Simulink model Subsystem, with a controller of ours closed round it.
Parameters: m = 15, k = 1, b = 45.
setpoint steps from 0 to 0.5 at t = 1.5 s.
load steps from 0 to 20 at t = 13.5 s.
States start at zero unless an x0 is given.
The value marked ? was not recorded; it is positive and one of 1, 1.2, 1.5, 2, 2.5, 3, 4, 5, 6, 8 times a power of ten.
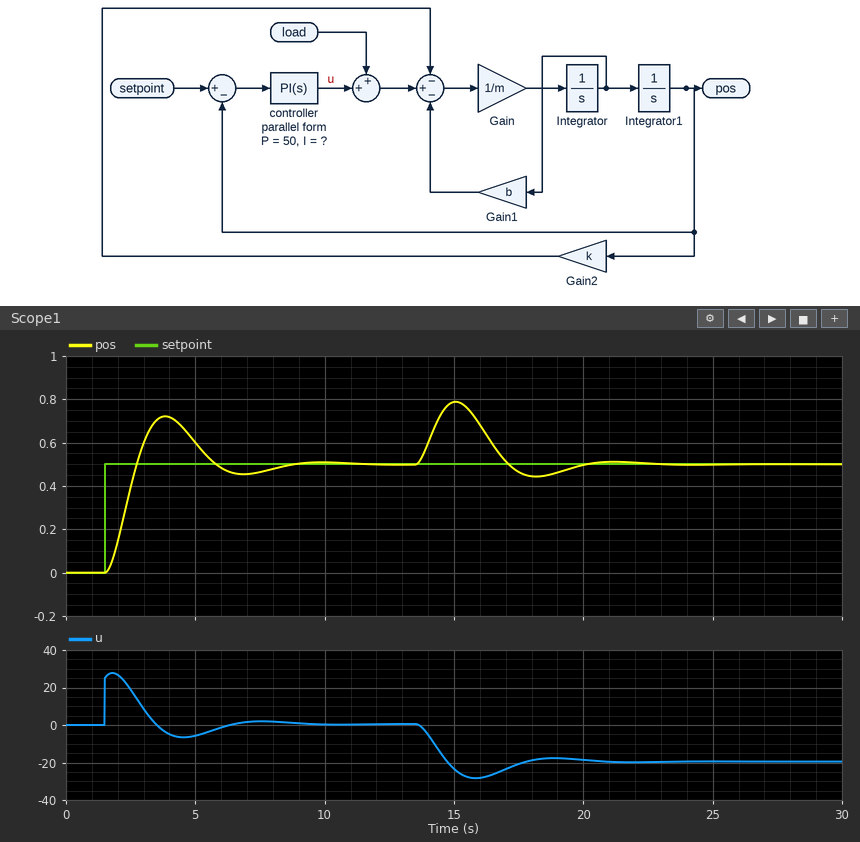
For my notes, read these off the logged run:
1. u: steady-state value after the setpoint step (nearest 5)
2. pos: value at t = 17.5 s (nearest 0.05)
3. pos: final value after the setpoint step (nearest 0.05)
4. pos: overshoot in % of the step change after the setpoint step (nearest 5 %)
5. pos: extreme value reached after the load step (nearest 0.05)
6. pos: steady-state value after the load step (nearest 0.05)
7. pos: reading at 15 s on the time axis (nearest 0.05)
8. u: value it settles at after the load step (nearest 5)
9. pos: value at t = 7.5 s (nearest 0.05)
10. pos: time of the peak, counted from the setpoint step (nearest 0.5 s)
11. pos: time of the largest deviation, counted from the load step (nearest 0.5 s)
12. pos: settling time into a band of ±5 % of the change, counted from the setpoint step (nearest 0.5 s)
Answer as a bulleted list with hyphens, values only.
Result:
- 0
- 0.45
- 0.50
- 45 %
- 0.80
- 0.50
- 0.80
- -20
- 0.45
- 2.5 s
- 1.5 s
- 6.5 s
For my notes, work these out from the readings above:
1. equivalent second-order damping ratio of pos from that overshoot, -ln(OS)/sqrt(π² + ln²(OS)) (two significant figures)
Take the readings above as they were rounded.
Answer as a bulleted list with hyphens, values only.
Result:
- 0.25
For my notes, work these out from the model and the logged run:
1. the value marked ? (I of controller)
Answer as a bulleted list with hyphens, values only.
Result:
- 40
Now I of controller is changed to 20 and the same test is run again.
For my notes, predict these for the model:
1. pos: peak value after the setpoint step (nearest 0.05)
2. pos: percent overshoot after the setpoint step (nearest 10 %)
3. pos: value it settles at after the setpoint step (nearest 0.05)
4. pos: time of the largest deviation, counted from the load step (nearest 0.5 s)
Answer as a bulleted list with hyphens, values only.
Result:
- 0.65
- 30 %
- 0.50
- 2.0 s
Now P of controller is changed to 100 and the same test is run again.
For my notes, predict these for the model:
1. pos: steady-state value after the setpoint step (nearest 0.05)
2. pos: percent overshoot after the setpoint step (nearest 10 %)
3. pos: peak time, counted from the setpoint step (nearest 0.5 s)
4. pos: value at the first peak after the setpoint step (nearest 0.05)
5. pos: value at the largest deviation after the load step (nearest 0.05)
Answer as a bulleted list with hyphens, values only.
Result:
- 0.50
- 30 %
- 1.5 s
- 0.65
- 0.70
